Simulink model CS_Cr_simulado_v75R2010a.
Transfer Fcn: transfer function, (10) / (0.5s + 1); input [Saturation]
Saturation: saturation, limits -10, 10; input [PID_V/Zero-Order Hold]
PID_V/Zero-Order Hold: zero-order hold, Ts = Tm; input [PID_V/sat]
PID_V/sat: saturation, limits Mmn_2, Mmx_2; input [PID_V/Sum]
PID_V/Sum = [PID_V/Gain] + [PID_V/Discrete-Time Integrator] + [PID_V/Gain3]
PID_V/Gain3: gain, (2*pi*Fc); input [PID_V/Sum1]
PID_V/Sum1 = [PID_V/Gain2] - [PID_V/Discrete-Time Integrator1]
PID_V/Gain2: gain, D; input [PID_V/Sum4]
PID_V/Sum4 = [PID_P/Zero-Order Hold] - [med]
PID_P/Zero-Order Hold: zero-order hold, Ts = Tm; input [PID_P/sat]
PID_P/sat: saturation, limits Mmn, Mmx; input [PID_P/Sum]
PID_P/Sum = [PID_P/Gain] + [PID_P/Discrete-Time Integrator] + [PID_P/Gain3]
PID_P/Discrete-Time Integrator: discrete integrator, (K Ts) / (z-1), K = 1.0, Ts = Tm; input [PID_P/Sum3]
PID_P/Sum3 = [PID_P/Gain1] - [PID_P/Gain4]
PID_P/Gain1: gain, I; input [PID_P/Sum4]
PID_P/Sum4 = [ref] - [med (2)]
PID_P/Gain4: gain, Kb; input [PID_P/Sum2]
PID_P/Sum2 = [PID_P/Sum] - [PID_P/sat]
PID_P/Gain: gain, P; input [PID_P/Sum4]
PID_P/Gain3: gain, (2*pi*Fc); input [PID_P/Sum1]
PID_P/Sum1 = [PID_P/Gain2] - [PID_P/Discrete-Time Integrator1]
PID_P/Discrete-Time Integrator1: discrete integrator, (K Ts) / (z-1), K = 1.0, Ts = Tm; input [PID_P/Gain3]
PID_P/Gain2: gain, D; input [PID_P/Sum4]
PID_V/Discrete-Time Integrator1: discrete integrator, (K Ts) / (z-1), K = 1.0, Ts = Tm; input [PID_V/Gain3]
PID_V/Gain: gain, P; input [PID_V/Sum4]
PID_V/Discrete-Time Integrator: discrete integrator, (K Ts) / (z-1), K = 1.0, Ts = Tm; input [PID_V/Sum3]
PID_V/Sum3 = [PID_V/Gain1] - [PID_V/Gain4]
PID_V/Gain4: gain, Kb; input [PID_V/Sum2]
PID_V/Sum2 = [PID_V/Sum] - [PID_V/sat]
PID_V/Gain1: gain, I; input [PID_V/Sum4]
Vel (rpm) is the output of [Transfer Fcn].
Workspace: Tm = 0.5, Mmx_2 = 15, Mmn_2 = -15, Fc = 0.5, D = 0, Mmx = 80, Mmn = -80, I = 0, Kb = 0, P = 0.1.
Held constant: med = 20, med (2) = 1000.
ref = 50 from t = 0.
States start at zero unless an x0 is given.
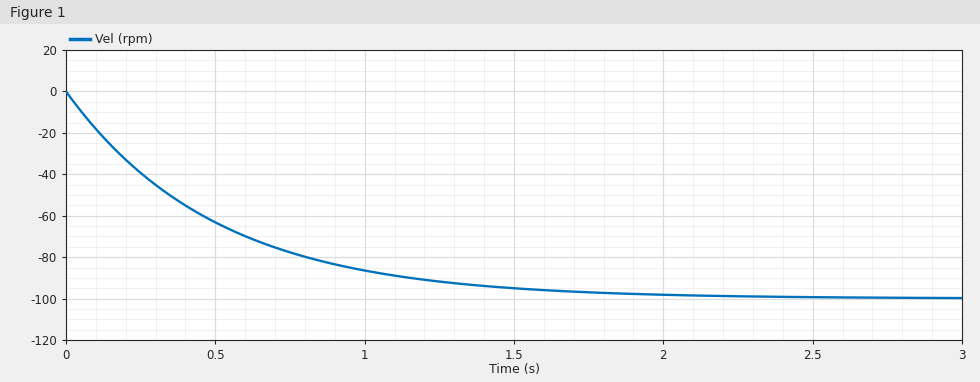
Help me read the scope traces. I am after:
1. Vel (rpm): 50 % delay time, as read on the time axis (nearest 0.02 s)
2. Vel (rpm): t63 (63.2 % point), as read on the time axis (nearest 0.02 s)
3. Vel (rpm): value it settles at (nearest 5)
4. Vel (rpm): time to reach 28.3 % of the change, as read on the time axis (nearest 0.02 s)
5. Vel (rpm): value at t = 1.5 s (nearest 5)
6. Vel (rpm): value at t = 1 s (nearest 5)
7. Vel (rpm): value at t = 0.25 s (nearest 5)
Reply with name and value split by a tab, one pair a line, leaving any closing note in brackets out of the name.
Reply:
Vel (rpm): 50 % delay time, as read on the time axis	0.34 s
Vel (rpm): t63 (63.2 % point), as read on the time axis	0.50 s
Vel (rpm): value it settles at	-100
Vel (rpm): time to reach 28.3 % of the change, as read on the time axis	0.16 s
Vel (rpm): value at t = 1.5 s	-95
Vel (rpm): value at t = 1 s	-85
Vel (rpm): value at t = 0.25 s	-40
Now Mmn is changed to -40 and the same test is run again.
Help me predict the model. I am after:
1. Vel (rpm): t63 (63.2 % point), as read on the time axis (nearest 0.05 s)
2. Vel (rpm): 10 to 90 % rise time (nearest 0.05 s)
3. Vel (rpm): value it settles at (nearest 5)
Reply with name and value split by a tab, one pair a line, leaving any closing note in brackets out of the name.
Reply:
Vel (rpm): t63 (63.2 % point), as read on the time axis	0.50 s
Vel (rpm): 10 to 90 % rise time	1.10 s
Vel (rpm): value it settles at	-60
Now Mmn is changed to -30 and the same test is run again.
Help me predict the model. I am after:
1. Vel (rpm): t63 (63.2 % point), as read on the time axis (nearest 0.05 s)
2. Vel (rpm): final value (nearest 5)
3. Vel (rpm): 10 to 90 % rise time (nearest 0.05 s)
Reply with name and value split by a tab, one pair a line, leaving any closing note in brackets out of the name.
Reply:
Vel (rpm): t63 (63.2 % point), as read on the time axis	0.50 s
Vel (rpm): final value	-50
Vel (rpm): 10 to 90 % rise time	1.10 s
